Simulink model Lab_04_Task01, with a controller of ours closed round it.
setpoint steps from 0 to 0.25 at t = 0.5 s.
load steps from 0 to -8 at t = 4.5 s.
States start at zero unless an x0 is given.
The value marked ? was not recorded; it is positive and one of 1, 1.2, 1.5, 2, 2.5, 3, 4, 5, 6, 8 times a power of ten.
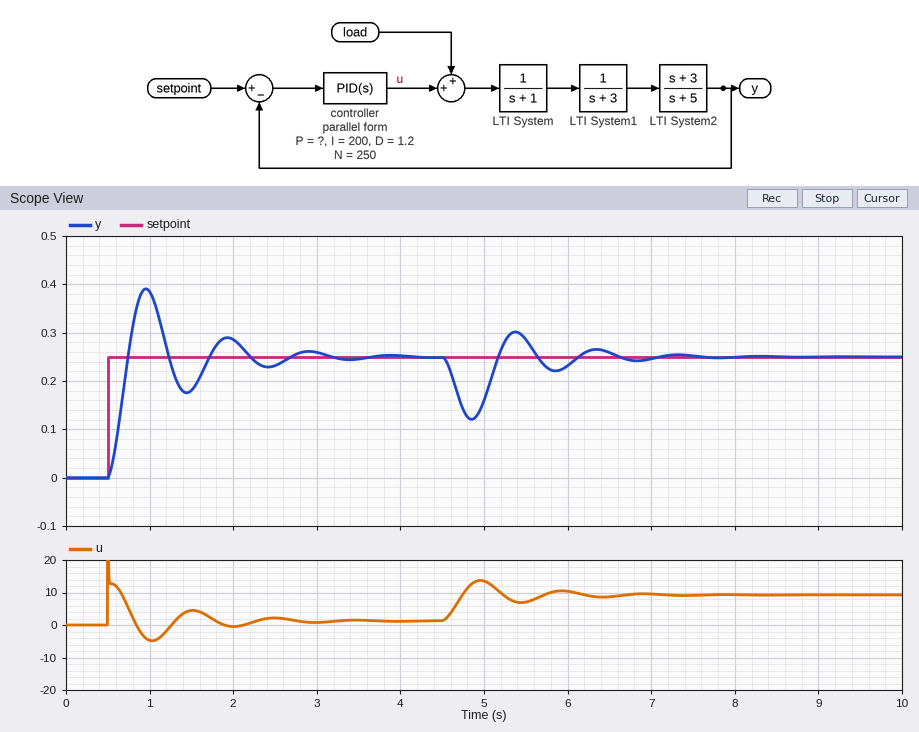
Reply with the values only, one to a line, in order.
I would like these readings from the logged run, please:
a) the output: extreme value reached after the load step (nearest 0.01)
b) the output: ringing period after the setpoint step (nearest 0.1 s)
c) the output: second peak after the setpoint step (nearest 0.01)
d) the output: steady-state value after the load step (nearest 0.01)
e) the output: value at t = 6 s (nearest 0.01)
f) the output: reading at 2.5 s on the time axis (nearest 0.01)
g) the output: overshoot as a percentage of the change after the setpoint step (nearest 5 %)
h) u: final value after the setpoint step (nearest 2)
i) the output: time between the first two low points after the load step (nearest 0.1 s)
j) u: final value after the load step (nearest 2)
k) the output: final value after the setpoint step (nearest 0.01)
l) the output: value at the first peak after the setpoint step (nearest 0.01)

0.12
1.0 s
0.29
0.25
0.23
0.23
55 %
2
1.0 s
10
0.25
0.39
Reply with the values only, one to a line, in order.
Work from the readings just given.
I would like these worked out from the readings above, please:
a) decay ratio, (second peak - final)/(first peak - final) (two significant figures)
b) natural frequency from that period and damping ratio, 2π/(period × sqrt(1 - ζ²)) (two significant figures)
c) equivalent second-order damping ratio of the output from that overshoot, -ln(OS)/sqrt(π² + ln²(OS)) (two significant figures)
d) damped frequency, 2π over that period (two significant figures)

0.29
6.4 rad/s
0.19
6.3 rad/s
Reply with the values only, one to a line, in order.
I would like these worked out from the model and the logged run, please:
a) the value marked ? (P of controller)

50
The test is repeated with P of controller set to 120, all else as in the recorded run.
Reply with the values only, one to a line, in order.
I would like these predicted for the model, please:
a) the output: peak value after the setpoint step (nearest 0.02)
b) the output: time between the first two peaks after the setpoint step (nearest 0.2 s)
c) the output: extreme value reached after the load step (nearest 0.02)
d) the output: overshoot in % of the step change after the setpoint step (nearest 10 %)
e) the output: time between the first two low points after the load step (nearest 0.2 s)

0.36
0.6 s
0.18
50 %
0.6 s
